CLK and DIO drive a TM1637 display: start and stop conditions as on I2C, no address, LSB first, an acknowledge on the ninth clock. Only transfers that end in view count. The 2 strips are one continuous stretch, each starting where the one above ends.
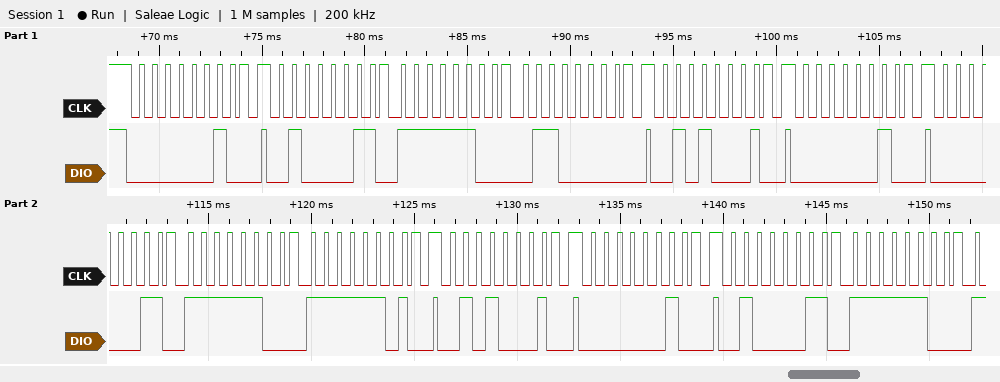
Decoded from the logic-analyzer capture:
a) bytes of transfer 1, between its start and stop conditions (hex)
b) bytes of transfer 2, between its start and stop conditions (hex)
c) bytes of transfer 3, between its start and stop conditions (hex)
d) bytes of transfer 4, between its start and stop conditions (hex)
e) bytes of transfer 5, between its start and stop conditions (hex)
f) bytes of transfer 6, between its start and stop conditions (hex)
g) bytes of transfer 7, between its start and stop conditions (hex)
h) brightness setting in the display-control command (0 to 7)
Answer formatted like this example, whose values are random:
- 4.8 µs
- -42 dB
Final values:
- 40
- C2 3F 06
- 8A
- 40
- C0 3F BF
- 8A
- 40
- 2
